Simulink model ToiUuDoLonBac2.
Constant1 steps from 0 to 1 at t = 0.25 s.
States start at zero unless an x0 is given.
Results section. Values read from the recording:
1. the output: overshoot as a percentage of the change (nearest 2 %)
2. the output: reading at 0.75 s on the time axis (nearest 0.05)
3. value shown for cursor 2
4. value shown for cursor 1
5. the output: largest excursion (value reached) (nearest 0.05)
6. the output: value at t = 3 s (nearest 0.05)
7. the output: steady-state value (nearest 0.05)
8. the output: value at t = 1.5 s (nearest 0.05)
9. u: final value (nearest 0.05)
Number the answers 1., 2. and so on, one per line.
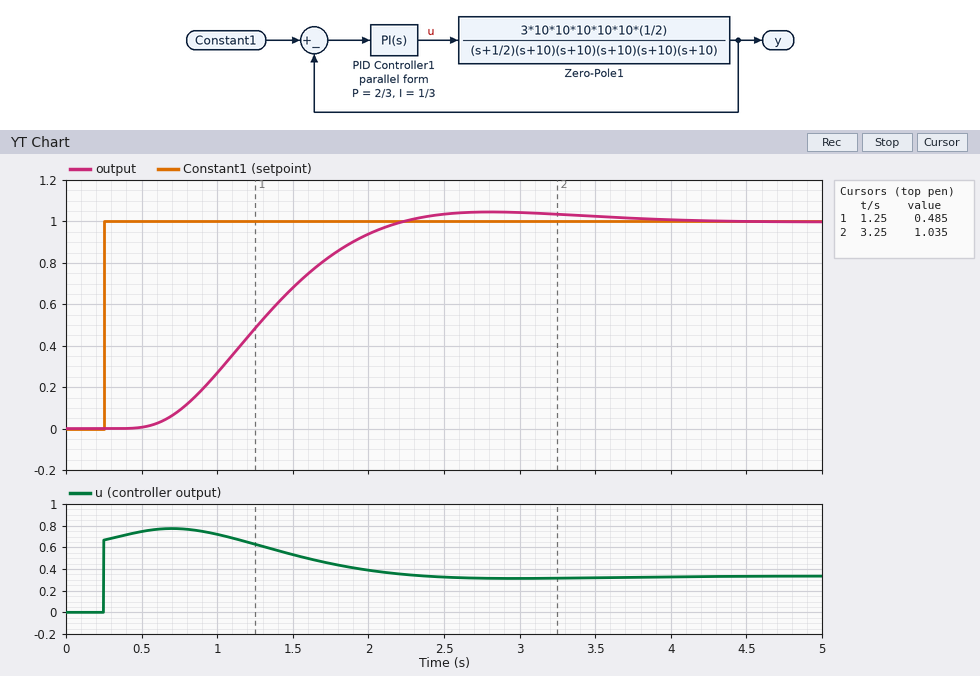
1. 4 %
2. 0.10
3. 1.035
4. 0.485
5. 1.05
6. 1.05
7. 1.00
8. 0.70
9. 0.35
